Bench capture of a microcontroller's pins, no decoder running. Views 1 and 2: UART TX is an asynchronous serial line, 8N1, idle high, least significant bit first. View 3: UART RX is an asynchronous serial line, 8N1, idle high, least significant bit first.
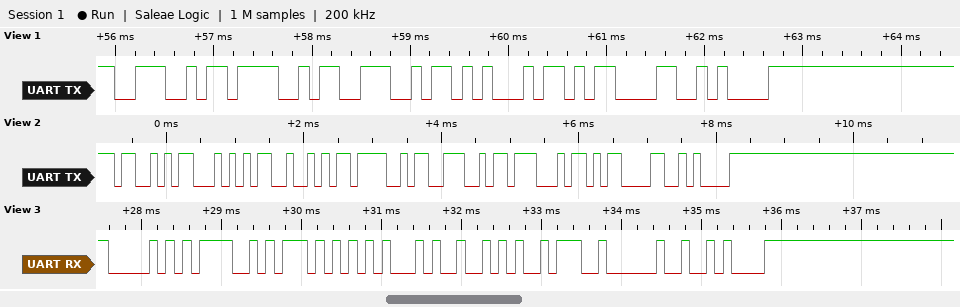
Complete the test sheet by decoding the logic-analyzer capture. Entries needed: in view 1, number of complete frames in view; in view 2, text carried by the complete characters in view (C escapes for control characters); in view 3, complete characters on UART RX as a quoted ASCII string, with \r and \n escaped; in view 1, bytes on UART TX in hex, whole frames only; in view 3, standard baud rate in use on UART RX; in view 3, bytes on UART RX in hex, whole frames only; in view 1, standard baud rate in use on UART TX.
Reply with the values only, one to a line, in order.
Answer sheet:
6
"STRONG\r\n"
"POWER: \n"
0x4E 0x4F 0x4E 0x45 0x0D 0x0A
9600 baud
50 4F 57 45 52 3A 20 0A
9600 baud
